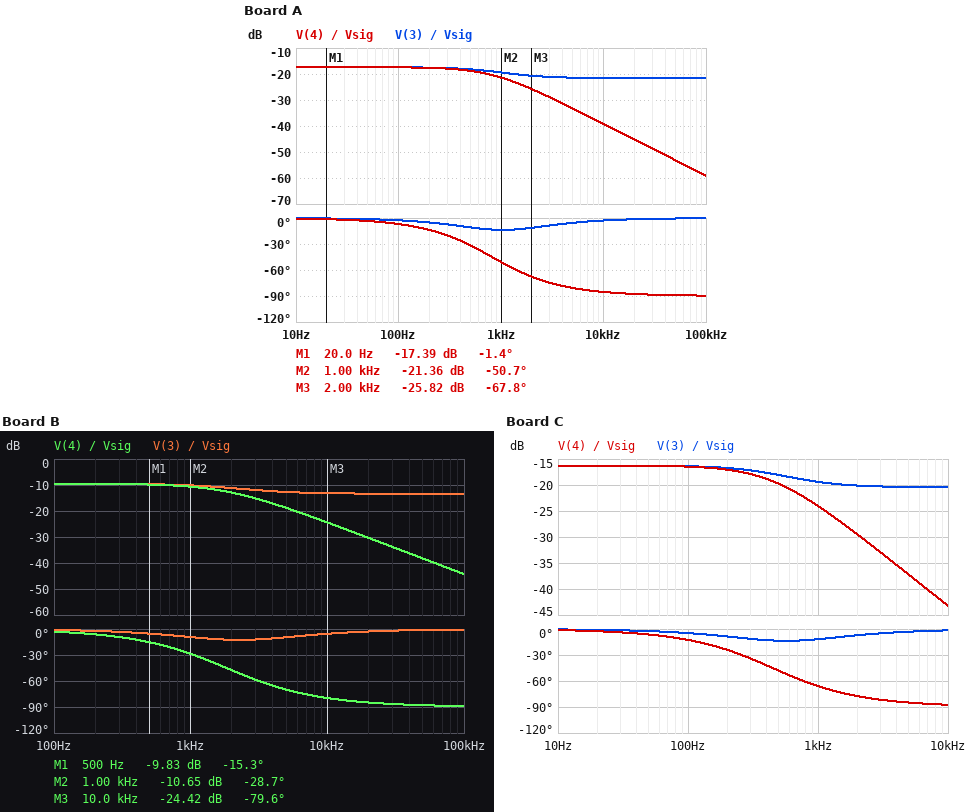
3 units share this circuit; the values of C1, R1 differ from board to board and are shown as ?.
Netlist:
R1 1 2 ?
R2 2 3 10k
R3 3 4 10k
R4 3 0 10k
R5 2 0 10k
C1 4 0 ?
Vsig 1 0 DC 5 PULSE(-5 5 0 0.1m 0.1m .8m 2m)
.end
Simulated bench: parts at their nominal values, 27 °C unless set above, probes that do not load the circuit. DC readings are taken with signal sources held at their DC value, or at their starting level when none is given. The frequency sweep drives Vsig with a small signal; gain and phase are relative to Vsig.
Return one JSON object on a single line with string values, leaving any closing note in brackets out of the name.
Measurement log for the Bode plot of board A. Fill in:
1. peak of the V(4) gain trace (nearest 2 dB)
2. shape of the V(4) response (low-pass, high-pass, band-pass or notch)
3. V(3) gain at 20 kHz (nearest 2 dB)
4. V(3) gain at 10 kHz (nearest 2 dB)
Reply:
{"peak of the V(4) gain trace": "-18 dB", "shape of the V(4) response": "low-pass", "V(3) gain at 20 kHz": "-22 dB", "V(3) gain at 10 kHz": "-22 dB"}
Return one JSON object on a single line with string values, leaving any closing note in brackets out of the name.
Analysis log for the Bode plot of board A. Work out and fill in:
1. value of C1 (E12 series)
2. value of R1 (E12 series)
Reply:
{"value of C1": "12 nF", "value of R1": "18 kΩ"}
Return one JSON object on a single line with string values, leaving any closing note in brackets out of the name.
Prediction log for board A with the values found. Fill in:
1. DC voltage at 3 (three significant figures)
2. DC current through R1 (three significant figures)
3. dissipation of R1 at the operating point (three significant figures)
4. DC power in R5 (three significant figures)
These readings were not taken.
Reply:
{"DC voltage at 3": "676 mV", "DC current through R1": "203 µA", "dissipation of R1 at the operating point": "740 µW", "DC power in R5": "183 µW"}
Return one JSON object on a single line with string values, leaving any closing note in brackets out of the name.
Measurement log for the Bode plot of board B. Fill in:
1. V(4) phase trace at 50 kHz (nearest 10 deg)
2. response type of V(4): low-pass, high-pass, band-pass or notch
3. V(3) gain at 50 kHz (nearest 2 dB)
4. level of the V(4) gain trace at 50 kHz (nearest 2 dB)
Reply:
{"V(4) phase trace at 50 kHz": "-90 deg", "response type of V(4): low-pass, high-pass, band-pass or notch": "low-pass", "V(3) gain at 50 kHz": "-14 dB", "level of the V(4) gain trace at 50 kHz": "-38 dB"}
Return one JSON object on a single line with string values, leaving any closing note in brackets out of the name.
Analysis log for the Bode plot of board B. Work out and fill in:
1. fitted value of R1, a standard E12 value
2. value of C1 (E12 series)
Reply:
{"fitted value of R1, a standard E12 value": "3.3 kΩ", "value of C1": "5.6 nF"}
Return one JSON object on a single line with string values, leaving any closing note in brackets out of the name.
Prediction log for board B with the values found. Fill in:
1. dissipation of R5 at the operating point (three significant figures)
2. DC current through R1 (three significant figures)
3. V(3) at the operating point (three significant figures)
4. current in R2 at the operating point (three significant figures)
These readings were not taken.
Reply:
{"dissipation of R5 at the operating point": "1.12 mW", "DC current through R1": "502 µA", "V(3) at the operating point": "1.67 V", "current in R2 at the operating point": "167 µA"}
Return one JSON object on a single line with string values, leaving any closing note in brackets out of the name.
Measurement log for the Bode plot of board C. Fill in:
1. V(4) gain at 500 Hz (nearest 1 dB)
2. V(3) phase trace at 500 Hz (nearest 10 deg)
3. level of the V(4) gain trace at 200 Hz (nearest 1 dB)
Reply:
{"V(4) gain at 500 Hz": "-20 dB", "V(3) phase trace at 500 Hz": "-10 deg", "level of the V(4) gain trace at 200 Hz": "-17 dB"}
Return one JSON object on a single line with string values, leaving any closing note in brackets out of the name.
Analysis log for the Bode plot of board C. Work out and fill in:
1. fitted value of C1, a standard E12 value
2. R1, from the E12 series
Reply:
{"fitted value of C1, a standard E12 value": "22 nF", "R1, from the E12 series": "15 kΩ"}
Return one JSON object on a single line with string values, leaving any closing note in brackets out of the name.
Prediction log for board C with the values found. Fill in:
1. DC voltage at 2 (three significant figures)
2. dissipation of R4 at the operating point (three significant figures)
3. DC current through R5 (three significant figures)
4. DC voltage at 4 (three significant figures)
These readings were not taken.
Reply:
{"DC voltage at 2": "1.54 V", "dissipation of R4 at the operating point": "59.2 µW", "DC current through R5": "154 µA", "DC voltage at 4": "769 mV"}
